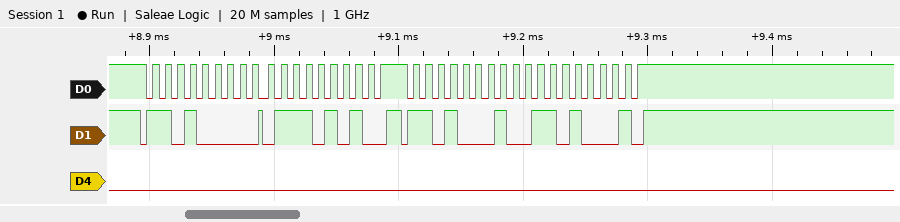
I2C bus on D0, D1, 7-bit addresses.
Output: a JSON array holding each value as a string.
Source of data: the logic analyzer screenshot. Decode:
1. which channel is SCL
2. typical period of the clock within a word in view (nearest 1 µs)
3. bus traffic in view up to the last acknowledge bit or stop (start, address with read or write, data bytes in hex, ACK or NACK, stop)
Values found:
["D0", "10 µs", "start, address 68 write ACK, 75 ACK, stop, start, address 68 read ACK, 68 NACK, stop"]
